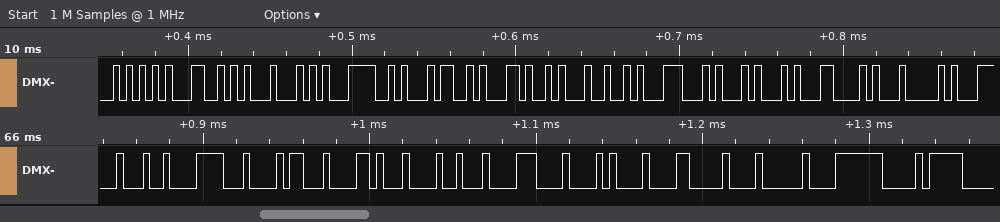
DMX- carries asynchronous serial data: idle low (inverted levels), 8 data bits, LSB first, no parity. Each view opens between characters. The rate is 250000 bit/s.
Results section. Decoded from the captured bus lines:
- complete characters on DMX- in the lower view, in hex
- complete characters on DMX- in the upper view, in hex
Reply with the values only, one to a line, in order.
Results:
B7, B8, B9, BA, BB, BC, BD, BE, BF, C0, C1
55, 56, 57, 58, 59, 5A, 5B, 5C, 5D, 5E, 5F
